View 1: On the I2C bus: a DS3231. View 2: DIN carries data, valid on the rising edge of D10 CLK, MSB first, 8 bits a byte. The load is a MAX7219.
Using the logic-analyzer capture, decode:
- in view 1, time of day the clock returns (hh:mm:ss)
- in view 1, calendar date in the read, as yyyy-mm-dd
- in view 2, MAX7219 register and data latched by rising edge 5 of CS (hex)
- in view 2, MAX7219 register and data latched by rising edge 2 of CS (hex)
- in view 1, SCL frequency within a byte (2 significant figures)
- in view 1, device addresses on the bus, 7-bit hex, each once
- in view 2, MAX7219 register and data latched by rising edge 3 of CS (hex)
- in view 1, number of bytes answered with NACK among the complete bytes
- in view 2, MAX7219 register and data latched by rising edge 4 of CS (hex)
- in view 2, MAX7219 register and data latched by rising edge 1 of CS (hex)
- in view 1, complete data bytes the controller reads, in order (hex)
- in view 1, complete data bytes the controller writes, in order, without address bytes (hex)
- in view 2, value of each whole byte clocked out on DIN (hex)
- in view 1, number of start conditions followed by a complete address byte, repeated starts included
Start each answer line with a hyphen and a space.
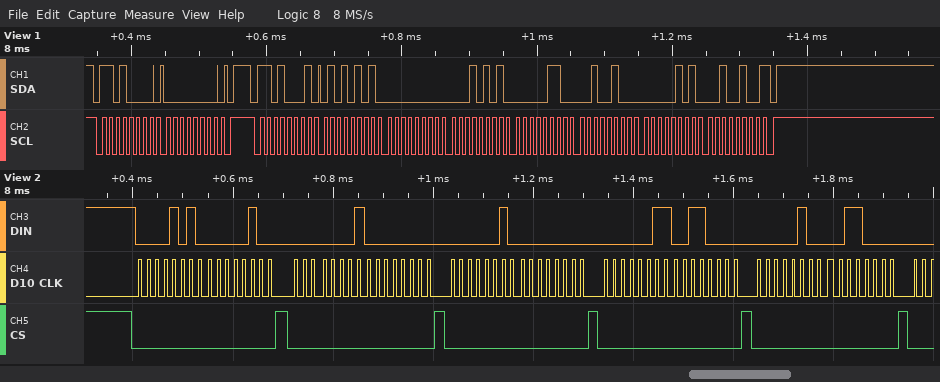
- 15:00:55
- 2024-05-24
- register 0x4, data 0x30
- register 0x1, data 0x00
- 100 kHz
- 0x68
- register 0x2, data 0x00
- 1
- register 0x3, data 0x30
- register 0xA, data 0x04
- 55 00 15 06 24 05 24
- 00
- 0A 04 01 00 02 00 03 30 04 30
- 2
